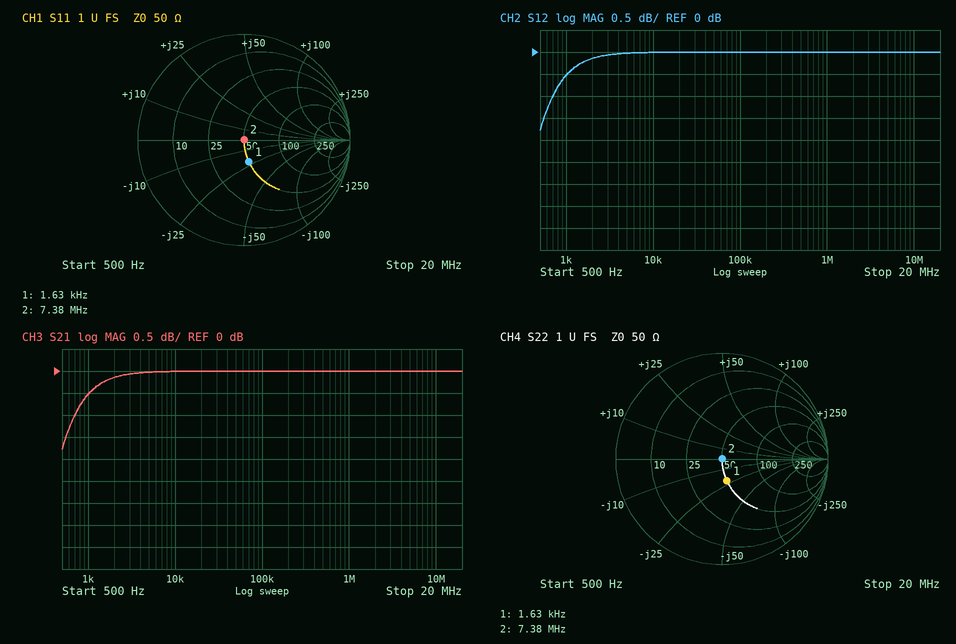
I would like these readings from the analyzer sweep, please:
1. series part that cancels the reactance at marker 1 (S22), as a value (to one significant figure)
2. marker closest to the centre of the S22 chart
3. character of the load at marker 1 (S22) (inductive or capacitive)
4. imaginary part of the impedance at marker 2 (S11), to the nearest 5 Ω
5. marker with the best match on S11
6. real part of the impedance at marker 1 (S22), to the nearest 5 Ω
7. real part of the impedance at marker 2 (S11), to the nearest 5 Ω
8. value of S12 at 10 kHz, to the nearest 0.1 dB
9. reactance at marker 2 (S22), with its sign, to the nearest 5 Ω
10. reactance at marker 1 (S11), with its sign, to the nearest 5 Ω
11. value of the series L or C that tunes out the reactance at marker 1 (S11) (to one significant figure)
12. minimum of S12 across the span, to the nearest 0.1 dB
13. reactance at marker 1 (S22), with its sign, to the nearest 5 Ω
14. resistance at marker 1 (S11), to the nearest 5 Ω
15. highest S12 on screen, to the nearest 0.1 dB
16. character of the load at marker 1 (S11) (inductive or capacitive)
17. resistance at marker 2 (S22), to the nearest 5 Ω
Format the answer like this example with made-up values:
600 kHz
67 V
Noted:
2 mH
marker 2
capacitive
0 Ω
marker 2
50 Ω
50 Ω
0.0 dB
0 Ω
-20 Ω
2 mH
-1.8 dB
-20 Ω
50 Ω
0.0 dB
capacitive
50 Ω
